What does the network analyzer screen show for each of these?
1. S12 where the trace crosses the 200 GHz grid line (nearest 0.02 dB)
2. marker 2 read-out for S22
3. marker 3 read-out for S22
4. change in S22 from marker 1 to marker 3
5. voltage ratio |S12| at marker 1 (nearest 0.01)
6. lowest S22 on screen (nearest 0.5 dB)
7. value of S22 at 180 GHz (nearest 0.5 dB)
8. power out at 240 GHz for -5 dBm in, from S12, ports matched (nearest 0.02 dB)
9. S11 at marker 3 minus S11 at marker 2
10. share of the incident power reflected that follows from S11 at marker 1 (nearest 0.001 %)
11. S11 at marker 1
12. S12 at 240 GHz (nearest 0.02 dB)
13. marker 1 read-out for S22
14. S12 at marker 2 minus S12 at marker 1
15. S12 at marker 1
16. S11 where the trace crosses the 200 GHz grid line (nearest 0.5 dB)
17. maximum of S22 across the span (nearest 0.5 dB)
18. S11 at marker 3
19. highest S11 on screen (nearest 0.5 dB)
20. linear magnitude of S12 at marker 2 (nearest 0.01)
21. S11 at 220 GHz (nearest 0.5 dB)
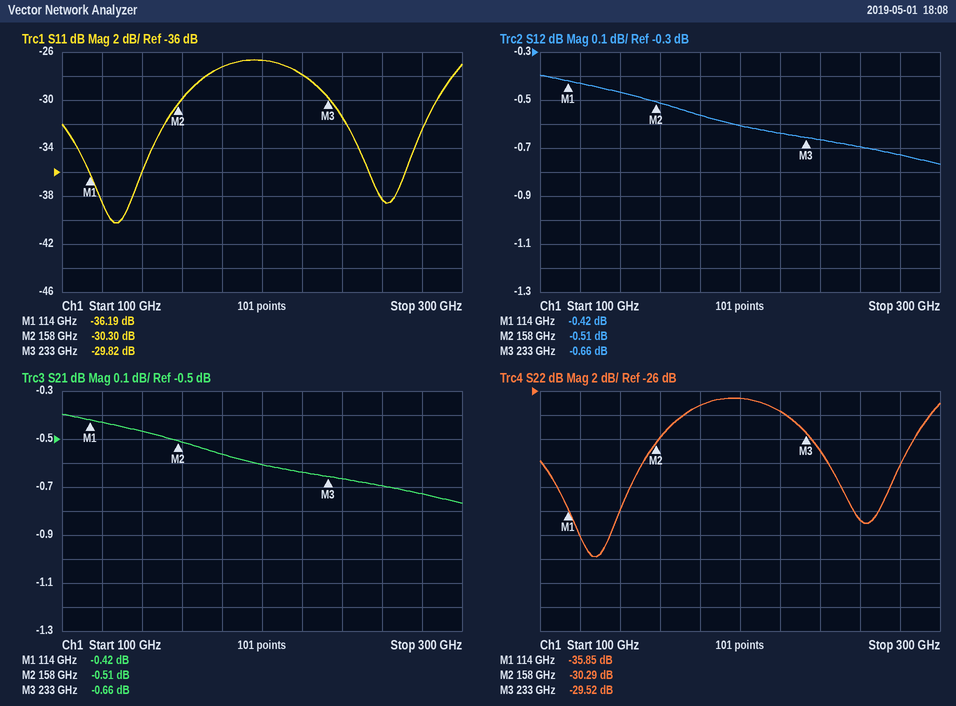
-0.60 dB
-30.29 dB
-29.52 dB
6.33 dB
0.95
-40.0 dB
-27.0 dB
-5.66 dBm
0.48 dB
0.024 %
-36.19 dB
-0.66 dB
-35.85 dB
-0.09 dB
-0.42 dB
-26.5 dB
-26.5 dB
-29.82 dB
-26.5 dB
0.94
-28.0 dB
